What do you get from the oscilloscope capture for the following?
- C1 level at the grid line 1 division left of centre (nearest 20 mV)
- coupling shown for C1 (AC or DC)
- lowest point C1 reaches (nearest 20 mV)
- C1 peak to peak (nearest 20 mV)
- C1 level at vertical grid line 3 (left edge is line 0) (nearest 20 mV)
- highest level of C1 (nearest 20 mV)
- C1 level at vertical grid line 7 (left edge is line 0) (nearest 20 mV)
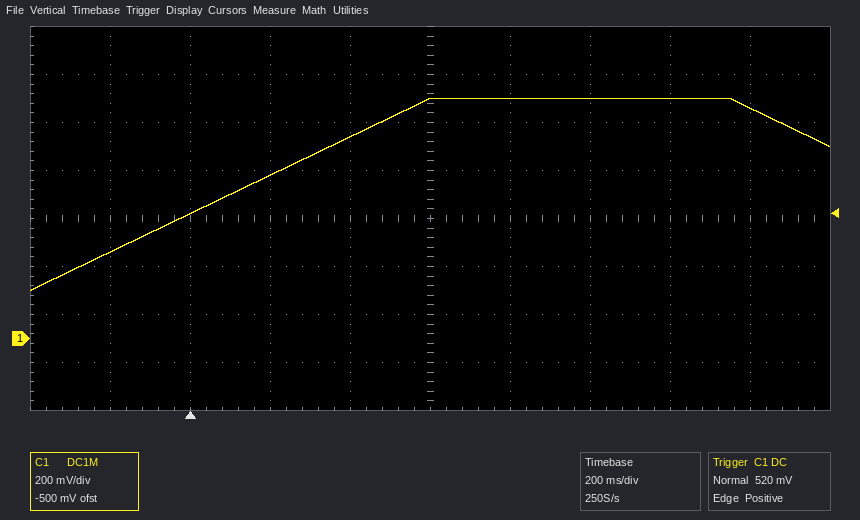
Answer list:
840 mV
DC
200 mV
800 mV
680 mV
1.00 V
1.00 V
